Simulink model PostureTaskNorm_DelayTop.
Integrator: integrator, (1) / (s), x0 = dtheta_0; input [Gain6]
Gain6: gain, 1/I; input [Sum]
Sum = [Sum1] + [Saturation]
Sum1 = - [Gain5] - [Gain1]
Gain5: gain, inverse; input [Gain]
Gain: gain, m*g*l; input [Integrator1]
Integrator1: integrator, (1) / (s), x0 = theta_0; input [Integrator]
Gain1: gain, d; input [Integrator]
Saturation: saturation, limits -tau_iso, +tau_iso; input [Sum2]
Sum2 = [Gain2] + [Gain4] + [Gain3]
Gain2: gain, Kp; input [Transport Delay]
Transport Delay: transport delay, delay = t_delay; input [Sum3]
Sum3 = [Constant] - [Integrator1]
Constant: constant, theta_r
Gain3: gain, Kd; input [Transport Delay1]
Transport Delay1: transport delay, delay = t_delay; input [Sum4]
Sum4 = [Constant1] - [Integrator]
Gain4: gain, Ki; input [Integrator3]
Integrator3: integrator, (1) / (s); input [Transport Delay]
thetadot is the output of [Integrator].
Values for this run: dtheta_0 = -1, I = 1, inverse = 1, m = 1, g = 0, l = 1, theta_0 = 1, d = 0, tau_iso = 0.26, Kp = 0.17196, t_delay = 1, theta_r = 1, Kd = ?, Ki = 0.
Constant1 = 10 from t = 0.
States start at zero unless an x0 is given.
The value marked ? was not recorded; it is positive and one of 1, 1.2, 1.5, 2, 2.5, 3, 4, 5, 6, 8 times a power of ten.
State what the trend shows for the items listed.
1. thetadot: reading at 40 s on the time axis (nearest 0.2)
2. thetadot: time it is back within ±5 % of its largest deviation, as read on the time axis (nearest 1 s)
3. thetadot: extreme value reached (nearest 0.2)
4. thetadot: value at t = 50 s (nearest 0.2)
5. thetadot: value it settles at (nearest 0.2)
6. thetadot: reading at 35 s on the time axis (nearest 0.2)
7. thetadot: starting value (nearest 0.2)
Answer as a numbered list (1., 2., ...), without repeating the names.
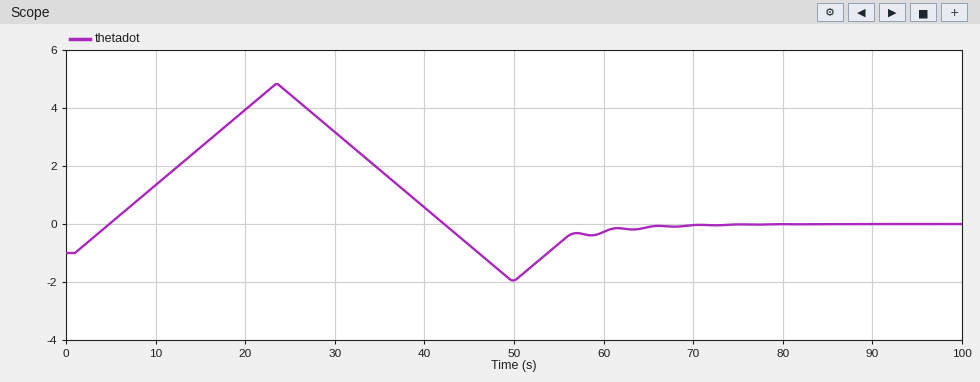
1. 0.6
2. 60 s
3. 4.8
4. -2.0
5. 0.0
6. 1.8
7. -1.0
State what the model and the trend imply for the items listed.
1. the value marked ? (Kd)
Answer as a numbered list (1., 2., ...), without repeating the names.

1. 1.2
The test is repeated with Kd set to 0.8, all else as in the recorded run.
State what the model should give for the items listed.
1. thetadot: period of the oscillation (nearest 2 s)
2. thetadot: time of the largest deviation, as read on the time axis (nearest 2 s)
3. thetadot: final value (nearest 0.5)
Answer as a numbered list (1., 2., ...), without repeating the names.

1. 40 s
2. 22 s
3. 0.0
